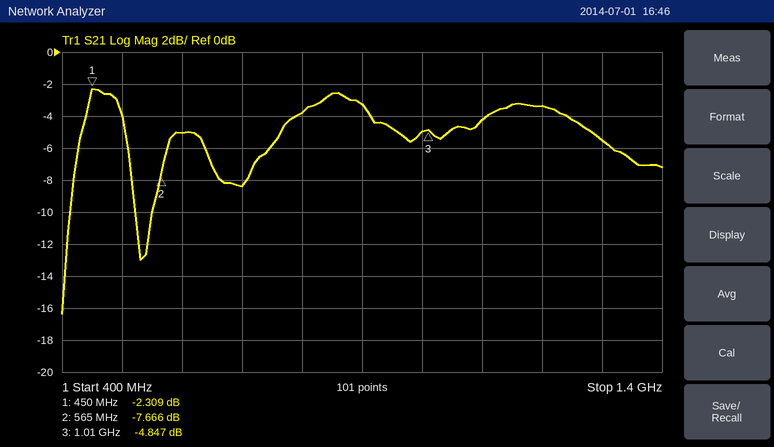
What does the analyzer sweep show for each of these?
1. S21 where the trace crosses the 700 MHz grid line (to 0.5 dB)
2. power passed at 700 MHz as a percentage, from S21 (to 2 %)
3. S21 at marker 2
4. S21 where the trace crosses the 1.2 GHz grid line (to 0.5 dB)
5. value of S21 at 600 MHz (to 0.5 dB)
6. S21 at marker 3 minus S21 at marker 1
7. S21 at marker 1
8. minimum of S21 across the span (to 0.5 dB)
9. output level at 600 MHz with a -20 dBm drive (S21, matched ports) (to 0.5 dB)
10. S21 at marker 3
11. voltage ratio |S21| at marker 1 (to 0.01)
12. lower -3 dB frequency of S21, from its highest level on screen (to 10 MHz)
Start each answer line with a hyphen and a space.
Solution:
- -8.5 dB
- 14 %
- -7.666 dB
- -3.5 dB
- -5.0 dB
- -2.538 dB
- -2.309 dB
- -16.5 dB
- -25.0 dBm
- -4.847 dB
- 0.77
- 430 MHz
